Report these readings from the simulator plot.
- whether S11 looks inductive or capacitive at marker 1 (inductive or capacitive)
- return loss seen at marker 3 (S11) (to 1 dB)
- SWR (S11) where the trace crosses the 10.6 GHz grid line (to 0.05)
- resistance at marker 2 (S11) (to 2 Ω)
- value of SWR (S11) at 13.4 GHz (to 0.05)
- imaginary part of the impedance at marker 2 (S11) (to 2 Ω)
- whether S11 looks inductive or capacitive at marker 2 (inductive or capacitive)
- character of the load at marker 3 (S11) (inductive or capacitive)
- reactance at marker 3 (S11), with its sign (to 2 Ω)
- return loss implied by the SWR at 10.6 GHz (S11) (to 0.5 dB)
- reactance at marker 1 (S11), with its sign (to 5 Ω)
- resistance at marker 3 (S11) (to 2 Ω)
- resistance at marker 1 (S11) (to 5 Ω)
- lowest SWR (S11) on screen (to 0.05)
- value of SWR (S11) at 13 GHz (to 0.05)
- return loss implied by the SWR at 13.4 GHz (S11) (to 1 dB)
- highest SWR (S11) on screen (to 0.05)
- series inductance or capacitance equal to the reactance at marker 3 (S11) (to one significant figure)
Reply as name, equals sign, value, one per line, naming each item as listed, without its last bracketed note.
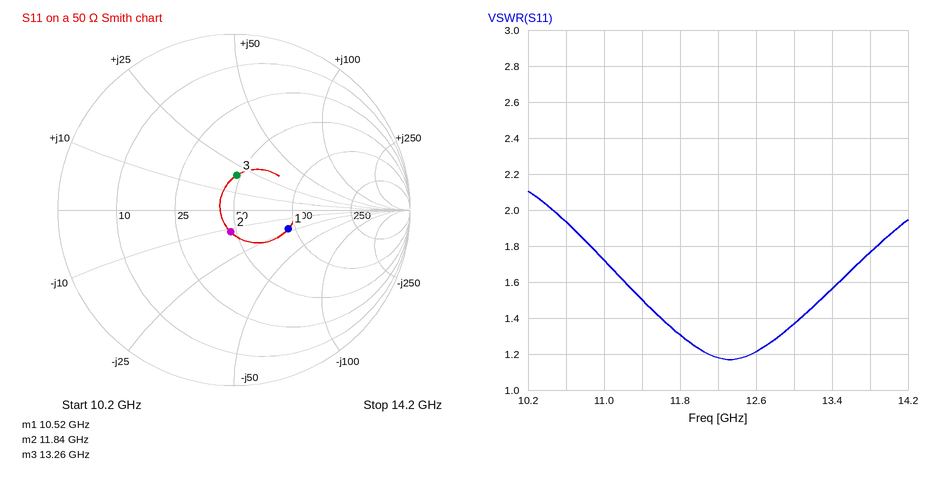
whether S11 looks inductive or capacitive at marker 1 = capacitive
return loss seen at marker 3 (S11) = 14 dB
SWR (S11) where the trace crosses the 10.6 GHz grid line = 1.95
resistance at marker 2 (S11) = 46 Ω
value of SWR (S11) at 13.4 GHz = 1.55
imaginary part of the impedance at marker 2 (S11) = -12 Ω
whether S11 looks inductive or capacitive at marker 2 = capacitive
character of the load at marker 3 (S11) = inductive
reactance at marker 3 (S11), with its sign = +20 Ω
return loss implied by the SWR at 10.6 GHz (S11) = 10.0 dB
reactance at marker 1 (S11), with its sign = -20 Ω
resistance at marker 3 (S11) = 48 Ω
resistance at marker 1 (S11) = 90 Ω
lowest SWR (S11) on screen = 1.15
value of SWR (S11) at 13 GHz = 1.35
return loss implied by the SWR at 13.4 GHz (S11) = 13 dB
highest SWR (S11) on screen = 2.10
series inductance or capacitance equal to the reactance at marker 3 (S11) = 200 pH
